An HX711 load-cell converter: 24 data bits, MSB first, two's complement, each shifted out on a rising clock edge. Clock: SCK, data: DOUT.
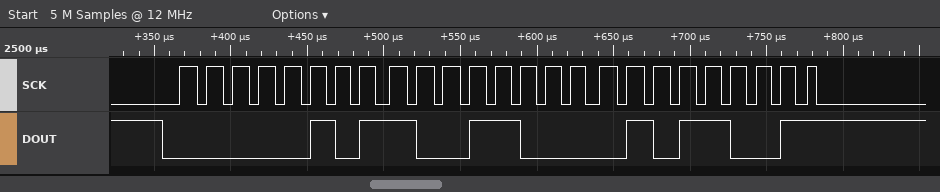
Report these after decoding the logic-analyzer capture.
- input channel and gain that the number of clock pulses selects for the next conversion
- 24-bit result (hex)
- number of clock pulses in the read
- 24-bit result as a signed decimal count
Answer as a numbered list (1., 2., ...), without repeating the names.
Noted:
1. channel A, gain 128
2. 0x059859
3. 25
4. 366681
